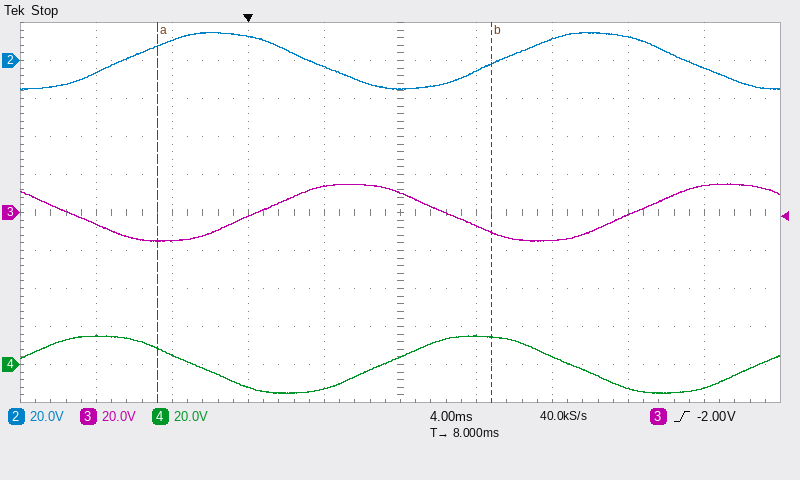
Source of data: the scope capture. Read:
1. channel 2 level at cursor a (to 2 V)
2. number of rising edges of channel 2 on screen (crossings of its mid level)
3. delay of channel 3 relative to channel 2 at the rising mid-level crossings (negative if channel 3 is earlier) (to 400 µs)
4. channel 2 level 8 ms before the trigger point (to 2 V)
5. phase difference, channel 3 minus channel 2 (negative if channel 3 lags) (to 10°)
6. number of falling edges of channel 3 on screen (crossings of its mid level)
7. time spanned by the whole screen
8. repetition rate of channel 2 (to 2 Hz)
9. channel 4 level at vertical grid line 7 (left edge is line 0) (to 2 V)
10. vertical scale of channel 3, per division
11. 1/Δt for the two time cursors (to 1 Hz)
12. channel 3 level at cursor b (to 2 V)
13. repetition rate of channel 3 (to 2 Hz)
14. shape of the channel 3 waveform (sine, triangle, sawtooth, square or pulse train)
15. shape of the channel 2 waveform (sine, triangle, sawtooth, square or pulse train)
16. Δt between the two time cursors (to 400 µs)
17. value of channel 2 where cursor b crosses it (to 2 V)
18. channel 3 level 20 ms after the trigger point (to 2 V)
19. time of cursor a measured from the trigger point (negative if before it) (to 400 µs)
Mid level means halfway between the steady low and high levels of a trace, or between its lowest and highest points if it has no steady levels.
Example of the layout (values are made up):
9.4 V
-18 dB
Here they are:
8 V
2
+7.2 ms
-6 V
-130°
2
40 ms
50 Hz
4 V
20 V
57 Hz
-10 V
50 Hz
sine
sine
17.6 ms
-2 V
-2 V
-4.8 ms
